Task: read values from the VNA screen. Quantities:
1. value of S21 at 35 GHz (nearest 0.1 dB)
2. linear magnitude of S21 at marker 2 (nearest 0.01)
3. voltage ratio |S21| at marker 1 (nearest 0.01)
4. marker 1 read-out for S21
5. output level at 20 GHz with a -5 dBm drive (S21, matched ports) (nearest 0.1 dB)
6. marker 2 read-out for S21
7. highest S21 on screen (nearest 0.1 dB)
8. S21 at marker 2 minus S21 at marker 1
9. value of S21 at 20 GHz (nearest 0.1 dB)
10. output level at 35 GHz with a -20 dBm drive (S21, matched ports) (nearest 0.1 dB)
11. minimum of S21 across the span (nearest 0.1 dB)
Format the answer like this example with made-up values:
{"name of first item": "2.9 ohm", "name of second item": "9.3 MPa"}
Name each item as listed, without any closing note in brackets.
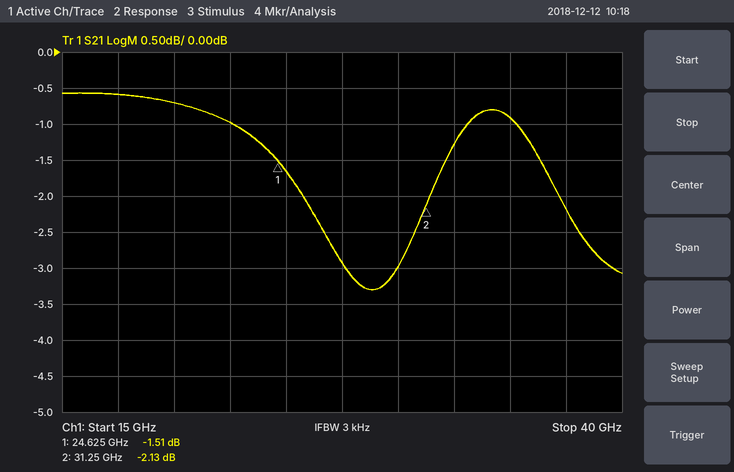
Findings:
{"value of S21 at 35 GHz": "-0.9 dB", "linear magnitude of S21 at marker 2": "0.78", "voltage ratio |S21| at marker 1": "0.84", "marker 1 read-out for S21": "-1.51 dB", "output level at 20 GHz with a -5 dBm drive (S21, matched ports)": "-5.7 dBm", "marker 2 read-out for S21": "-2.13 dB", "highest S21 on screen": "-0.6 dB", "S21 at marker 2 minus S21 at marker 1": "-0.62 dB", "value of S21 at 20 GHz": "-0.7 dB", "output level at 35 GHz with a -20 dBm drive (S21, matched ports)": "-20.9 dBm", "minimum of S21 across the span": "-3.3 dB"}
